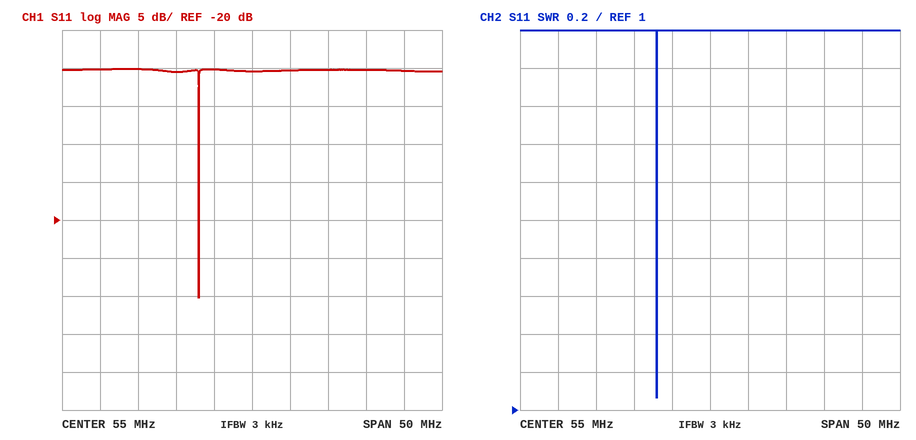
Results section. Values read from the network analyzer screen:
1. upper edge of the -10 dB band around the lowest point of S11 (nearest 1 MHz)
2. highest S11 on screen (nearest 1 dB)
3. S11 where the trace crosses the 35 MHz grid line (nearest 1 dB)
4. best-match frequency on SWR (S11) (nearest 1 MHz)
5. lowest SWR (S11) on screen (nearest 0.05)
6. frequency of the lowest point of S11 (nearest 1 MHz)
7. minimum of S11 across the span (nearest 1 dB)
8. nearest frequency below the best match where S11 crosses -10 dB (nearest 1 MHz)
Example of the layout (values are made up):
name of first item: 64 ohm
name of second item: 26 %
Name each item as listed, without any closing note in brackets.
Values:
upper edge of the -10 dB band around the lowest point of S11: 48 MHz
highest S11 on screen: 0 dB
S11 where the trace crosses the 35 MHz grid line: 0 dB
best-match frequency on SWR (S11): 48 MHz
lowest SWR (S11) on screen: 1.05
frequency of the lowest point of S11: 48 MHz
minimum of S11 across the span: -30 dB
nearest frequency below the best match where S11 crosses -10 dB: 48 MHz
